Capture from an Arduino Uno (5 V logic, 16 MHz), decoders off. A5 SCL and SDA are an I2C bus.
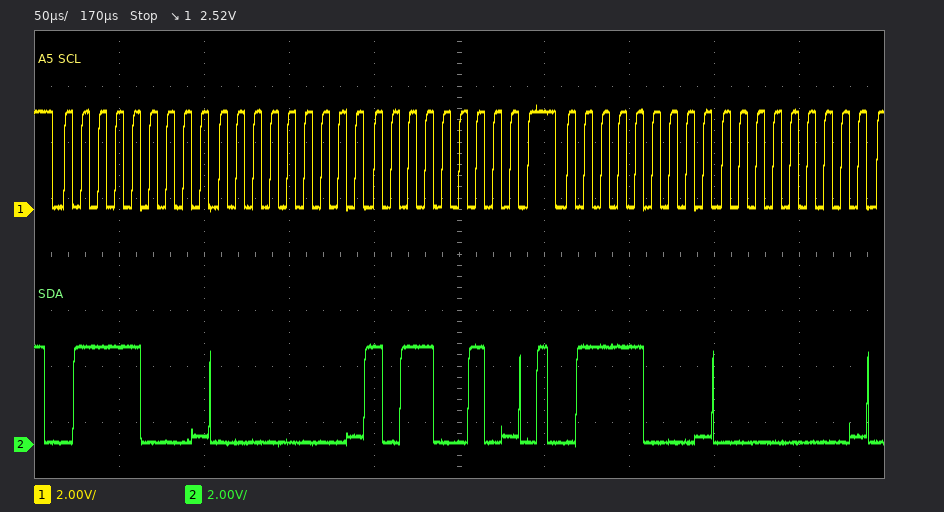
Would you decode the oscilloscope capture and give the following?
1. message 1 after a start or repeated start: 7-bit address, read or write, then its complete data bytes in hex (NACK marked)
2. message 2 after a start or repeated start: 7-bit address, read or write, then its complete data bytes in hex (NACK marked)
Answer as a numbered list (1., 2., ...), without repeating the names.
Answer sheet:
1. 0x3C write: 00 B2
2. 0x3C write: 00
